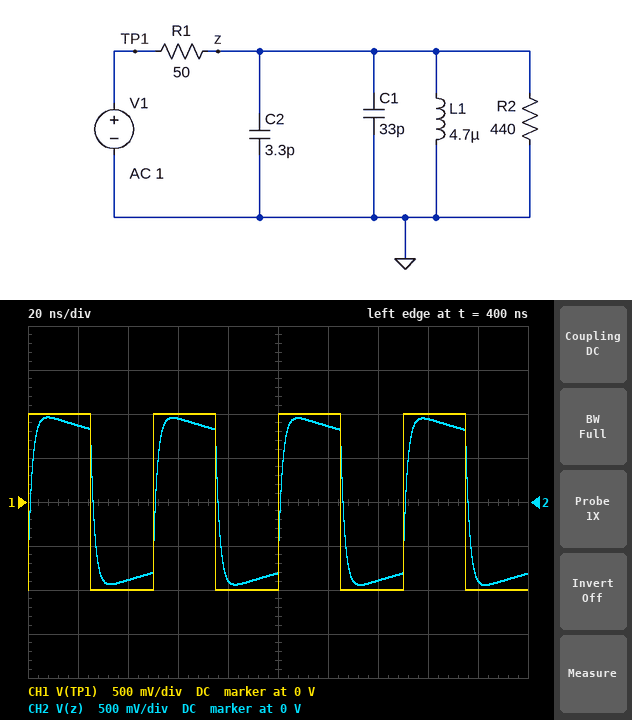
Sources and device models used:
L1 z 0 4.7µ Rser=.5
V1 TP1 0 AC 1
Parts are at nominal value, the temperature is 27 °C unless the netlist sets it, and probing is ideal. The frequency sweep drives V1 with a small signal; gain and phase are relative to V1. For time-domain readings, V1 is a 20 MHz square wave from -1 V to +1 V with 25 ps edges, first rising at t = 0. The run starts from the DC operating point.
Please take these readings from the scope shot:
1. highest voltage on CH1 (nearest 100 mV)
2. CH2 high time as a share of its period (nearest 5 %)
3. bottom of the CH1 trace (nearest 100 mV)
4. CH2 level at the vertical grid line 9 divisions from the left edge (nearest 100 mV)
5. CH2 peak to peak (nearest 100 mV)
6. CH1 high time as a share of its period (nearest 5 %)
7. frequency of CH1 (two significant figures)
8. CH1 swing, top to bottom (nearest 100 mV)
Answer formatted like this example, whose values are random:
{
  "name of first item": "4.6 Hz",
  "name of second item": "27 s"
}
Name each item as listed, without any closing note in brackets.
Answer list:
{
  "highest voltage on CH1": "1.0 V",
  "CH2 high time as a share of its period": "50 %",
  "bottom of the CH1 trace": "-1.0 V",
  "CH2 level at the vertical grid line 9 divisions from the left edge": "-900 mV",
  "CH2 peak to peak": "1.9 V",
  "CH1 high time as a share of its period": "50 %",
  "frequency of CH1": "20 MHz",
  "CH1 swing, top to bottom": "2.0 V"
}
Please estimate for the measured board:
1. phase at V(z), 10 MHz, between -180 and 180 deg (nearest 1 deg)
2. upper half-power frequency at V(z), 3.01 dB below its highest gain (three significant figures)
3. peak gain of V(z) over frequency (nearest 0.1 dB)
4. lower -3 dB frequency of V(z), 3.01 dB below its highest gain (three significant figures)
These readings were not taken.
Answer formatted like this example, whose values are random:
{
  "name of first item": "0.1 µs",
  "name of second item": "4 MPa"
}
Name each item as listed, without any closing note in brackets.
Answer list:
{
  "phase at V(z), 10 MHz, between -180 and 180 deg": "3 deg",
  "upper half-power frequency at V(z), 3.01 dB below its highest gain": "99.2 MHz",
  "peak gain of V(z) over frequency": "-0.9 dB",
  "lower -3 dB frequency of V(z), 3.01 dB below its highest gain": "1.51 MHz"
}
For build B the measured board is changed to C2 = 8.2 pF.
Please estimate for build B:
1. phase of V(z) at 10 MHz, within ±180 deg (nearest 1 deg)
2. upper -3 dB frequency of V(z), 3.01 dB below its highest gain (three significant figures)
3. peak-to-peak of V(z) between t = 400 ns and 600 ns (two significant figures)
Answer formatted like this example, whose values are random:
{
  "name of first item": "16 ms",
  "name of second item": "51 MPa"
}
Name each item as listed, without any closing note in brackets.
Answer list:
{
  "phase of V(z) at 10 MHz, within ±180 deg": "2 deg",
  "upper -3 dB frequency of V(z), 3.01 dB below its highest gain": "87.6 MHz",
  "peak-to-peak of V(z) between t = 400 ns and 600 ns": "1.9 V"
}
